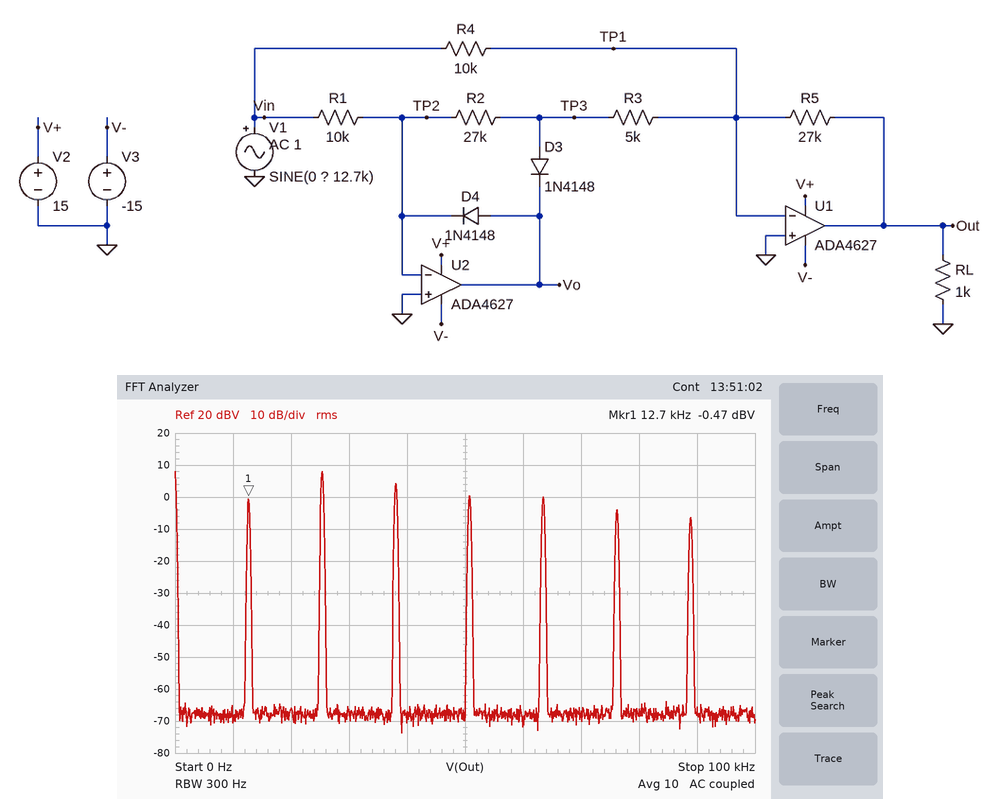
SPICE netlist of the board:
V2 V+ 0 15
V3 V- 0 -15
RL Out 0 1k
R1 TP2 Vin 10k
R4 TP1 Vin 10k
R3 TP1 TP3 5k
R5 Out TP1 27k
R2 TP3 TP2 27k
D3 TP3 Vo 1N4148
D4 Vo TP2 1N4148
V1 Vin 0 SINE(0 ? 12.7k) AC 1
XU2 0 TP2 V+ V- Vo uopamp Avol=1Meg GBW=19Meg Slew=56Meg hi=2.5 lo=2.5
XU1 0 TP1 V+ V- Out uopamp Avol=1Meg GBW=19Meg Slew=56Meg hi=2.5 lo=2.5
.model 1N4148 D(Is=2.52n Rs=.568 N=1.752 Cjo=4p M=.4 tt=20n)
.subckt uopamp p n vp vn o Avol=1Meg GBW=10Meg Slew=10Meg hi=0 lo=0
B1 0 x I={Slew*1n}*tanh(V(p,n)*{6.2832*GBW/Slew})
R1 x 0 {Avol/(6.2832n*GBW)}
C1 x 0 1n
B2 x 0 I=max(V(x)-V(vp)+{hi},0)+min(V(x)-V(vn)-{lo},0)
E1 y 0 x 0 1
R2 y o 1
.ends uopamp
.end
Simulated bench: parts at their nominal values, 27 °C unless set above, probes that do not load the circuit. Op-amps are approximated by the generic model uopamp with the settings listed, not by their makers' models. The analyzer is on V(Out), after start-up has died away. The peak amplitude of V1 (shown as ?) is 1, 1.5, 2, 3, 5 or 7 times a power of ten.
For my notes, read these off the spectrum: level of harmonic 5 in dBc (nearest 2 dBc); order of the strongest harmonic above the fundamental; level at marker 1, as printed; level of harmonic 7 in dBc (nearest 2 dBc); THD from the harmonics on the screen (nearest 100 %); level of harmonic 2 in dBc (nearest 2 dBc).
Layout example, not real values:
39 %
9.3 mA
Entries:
0 dBc
2
-0.47 dBV
-6 dBc
400 %
8 dBc
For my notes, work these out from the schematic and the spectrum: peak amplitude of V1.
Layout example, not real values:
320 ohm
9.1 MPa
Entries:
5 V
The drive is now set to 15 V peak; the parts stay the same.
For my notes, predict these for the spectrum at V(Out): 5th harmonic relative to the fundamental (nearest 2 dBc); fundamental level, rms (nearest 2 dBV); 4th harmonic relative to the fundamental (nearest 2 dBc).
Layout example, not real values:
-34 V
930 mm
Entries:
10 dBc
-18 dBV
18 dBc
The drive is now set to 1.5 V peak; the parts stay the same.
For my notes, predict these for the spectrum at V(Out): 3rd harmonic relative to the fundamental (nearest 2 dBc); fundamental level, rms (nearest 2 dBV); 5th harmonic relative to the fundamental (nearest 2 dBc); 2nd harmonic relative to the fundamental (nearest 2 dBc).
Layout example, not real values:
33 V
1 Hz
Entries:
-14 dBc
12 dBV
-30 dBc
-4 dBc
